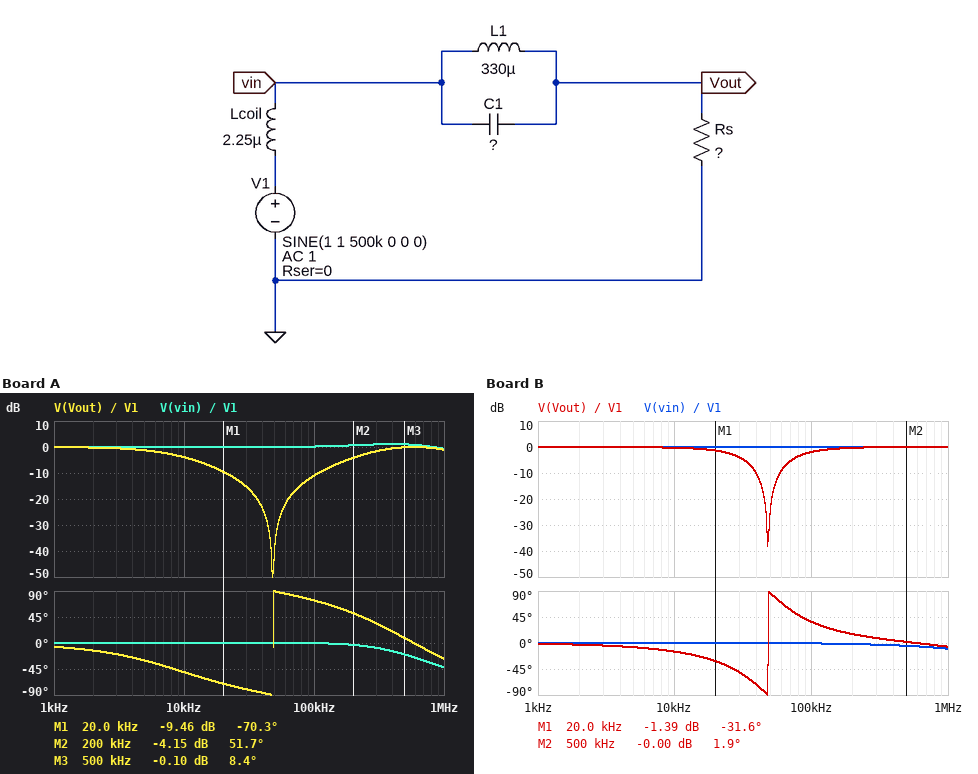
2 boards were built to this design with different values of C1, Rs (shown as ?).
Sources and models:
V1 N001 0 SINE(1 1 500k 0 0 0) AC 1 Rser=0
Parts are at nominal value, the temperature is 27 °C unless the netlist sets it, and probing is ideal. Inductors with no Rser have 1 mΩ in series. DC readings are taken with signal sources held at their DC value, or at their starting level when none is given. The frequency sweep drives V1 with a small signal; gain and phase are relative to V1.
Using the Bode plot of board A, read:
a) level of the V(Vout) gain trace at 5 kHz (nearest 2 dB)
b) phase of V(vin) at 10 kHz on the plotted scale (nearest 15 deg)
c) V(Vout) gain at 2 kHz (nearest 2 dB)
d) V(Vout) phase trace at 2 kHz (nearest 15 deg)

-2 dB
0 deg
0 dB
-15 deg
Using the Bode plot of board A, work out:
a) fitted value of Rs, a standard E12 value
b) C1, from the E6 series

18 Ω
33 nF
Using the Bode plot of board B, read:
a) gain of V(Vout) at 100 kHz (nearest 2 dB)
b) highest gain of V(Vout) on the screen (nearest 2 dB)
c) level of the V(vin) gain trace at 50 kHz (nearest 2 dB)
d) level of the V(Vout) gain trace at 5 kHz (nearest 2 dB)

-2 dB
0 dB
0 dB
0 dB
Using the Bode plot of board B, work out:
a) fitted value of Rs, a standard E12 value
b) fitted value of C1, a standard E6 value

82 Ω
33 nF
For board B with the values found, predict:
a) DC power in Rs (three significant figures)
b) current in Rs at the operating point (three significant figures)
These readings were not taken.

12.2 mW
12.2 mA
